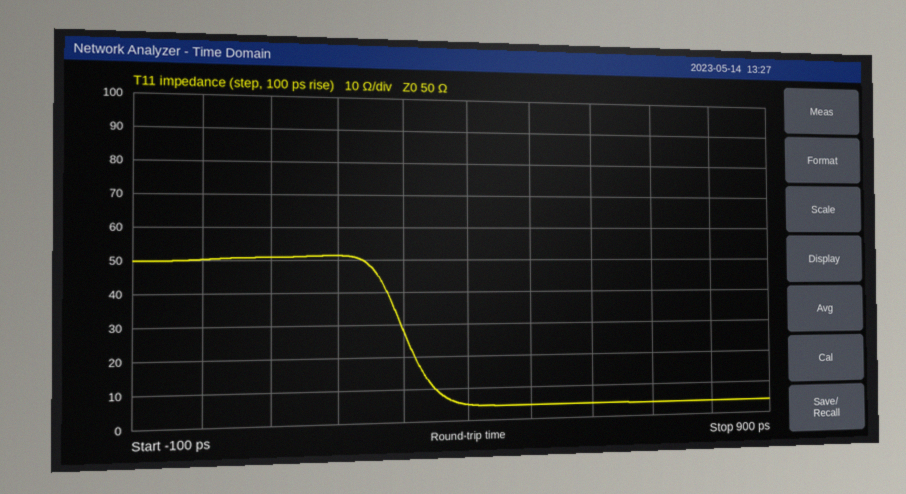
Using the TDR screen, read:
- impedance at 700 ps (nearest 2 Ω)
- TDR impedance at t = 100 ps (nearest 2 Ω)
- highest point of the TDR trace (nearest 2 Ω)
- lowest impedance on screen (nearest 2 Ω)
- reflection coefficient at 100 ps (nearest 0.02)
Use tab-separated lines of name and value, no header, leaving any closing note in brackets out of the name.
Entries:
impedance at 700 ps	4 Ω
TDR impedance at t = 100 ps	50 Ω
highest point of the TDR trace	52 Ω
lowest impedance on screen	4 Ω
reflection coefficient at 100 ps	0.00
